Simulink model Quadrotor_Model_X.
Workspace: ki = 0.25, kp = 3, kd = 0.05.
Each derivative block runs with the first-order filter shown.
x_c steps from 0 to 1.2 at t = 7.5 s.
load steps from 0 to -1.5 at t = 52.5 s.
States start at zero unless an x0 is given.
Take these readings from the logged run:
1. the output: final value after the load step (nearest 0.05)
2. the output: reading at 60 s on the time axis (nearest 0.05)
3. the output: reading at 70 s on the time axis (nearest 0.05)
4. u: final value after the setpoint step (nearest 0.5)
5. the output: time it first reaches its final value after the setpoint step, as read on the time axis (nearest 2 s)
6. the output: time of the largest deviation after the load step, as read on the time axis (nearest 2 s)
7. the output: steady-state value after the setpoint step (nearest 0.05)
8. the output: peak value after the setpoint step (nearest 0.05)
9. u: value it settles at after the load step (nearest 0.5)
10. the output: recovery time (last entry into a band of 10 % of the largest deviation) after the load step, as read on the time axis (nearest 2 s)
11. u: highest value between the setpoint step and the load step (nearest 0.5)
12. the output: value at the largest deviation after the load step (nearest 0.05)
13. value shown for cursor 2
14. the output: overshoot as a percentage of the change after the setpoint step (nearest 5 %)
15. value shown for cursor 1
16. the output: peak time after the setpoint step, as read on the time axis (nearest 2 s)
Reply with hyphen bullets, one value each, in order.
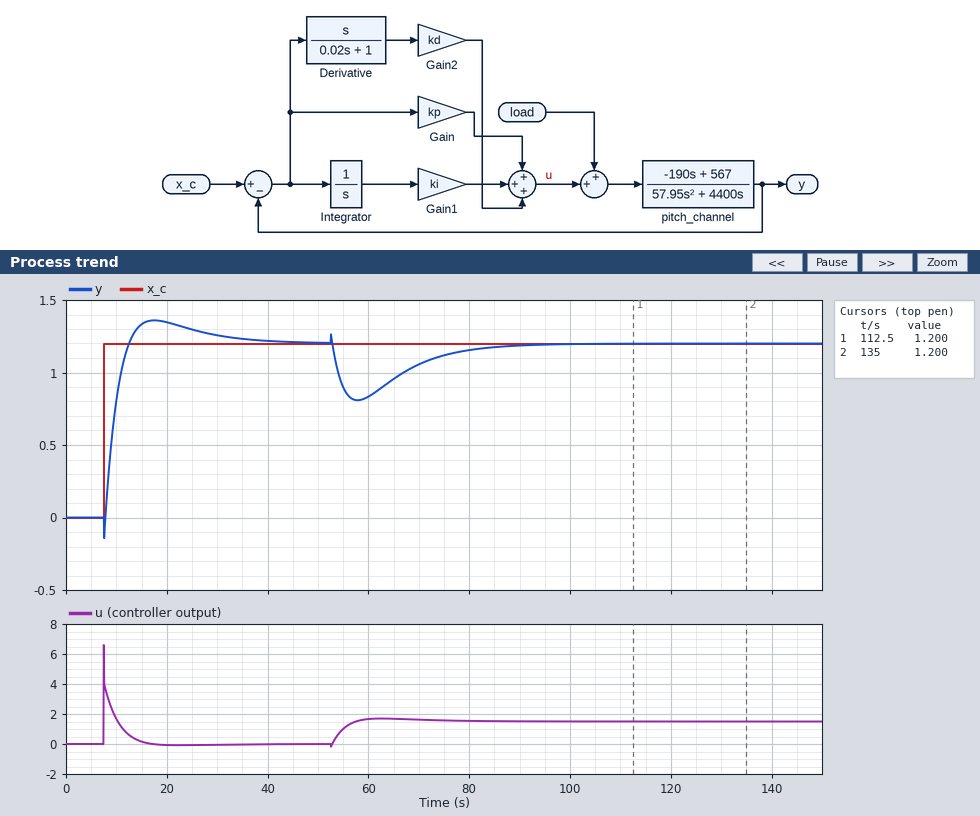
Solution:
- 1.20
- 0.85
- 1.05
- 0.0
- 12 s
- 58 s
- 1.20
- 1.35
- 1.5
- 82 s
- 6.5
- 0.80
- 1.200
- 15 %
- 1.200
- 18 s
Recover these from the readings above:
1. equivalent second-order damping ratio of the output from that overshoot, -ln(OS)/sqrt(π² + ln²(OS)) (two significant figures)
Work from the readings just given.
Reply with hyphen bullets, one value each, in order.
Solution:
- 0.52
